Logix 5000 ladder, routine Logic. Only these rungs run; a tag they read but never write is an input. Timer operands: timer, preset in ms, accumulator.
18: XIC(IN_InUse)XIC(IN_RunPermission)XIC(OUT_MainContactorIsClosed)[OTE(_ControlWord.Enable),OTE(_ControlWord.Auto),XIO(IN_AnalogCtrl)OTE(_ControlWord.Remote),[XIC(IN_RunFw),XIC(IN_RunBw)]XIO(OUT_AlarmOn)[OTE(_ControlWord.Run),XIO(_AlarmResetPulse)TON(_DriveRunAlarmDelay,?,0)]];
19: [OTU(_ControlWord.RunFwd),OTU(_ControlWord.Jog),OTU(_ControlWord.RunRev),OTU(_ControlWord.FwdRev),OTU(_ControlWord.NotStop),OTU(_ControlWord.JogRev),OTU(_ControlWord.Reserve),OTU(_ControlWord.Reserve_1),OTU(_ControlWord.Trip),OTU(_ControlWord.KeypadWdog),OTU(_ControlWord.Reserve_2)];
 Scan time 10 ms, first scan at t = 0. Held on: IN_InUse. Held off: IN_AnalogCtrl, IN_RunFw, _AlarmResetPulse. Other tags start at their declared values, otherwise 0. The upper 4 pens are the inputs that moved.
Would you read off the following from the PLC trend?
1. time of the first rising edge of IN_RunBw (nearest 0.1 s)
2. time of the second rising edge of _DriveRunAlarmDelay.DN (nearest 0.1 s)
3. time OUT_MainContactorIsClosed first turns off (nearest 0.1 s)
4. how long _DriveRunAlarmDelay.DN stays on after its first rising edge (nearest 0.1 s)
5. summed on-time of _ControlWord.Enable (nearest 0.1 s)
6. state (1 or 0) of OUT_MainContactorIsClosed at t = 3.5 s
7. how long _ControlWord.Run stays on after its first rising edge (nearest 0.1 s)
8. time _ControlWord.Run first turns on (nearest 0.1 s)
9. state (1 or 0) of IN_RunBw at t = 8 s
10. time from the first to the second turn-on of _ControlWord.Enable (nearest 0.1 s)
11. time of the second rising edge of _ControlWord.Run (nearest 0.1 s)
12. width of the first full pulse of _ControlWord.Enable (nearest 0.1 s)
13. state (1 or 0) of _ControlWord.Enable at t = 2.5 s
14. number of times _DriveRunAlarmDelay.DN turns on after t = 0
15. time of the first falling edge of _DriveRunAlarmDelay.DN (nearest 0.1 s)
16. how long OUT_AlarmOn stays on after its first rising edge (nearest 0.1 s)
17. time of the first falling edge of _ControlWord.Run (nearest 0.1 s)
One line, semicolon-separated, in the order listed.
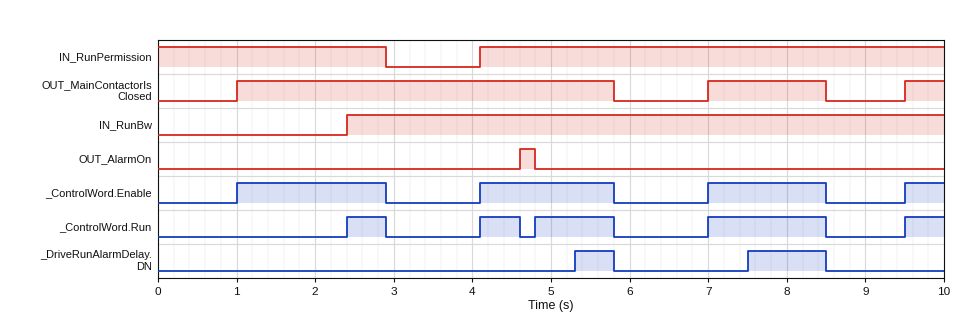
2.4 s; 7.5 s; 5.8 s; 0.5 s; 5.6 s; 1; 0.5 s; 2.4 s; 1; 3.1 s; 4.1 s; 1.9 s; 1; 2; 5.8 s; 0.2 s; 2.9 s
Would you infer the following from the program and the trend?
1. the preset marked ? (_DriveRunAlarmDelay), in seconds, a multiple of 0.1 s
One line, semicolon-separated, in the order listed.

0.5 s
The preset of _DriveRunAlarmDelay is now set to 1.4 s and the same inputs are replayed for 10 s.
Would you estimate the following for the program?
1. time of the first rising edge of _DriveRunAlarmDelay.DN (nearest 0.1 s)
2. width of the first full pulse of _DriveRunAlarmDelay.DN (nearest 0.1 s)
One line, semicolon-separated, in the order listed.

8.4 s; 0.1 s
